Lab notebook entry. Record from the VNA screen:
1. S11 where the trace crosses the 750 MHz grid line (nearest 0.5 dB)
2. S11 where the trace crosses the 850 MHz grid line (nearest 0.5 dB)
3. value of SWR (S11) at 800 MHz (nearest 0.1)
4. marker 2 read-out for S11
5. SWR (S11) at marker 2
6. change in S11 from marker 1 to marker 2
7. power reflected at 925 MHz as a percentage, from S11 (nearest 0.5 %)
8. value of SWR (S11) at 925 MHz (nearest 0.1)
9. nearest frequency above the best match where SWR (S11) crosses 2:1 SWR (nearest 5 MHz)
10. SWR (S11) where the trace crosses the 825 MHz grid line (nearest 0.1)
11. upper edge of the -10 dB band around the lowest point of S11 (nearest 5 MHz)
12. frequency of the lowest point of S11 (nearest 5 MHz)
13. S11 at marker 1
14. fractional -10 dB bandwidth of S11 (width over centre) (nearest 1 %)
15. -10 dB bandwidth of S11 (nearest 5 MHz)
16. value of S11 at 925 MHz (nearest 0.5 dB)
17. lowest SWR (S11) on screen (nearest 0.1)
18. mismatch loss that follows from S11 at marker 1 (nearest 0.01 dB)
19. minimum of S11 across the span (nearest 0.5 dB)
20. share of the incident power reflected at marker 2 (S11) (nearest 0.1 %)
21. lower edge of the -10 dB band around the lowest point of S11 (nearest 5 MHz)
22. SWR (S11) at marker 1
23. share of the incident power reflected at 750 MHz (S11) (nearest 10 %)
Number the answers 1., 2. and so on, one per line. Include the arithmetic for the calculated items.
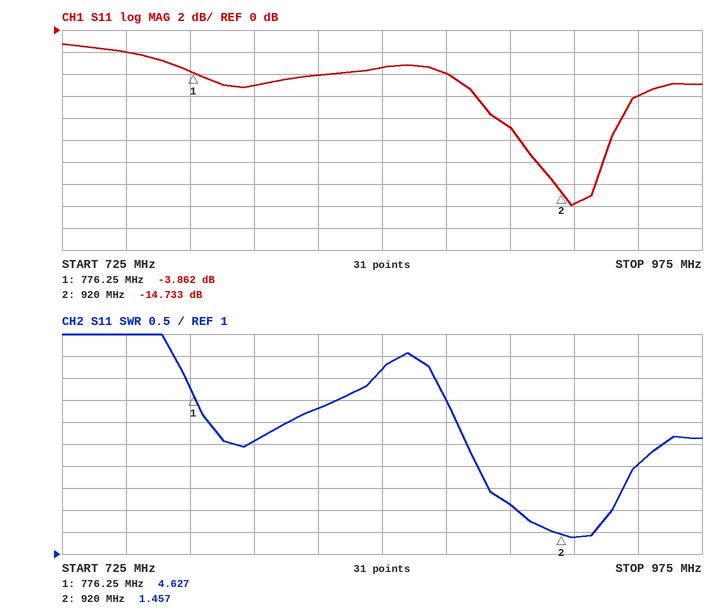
1. -2.0 dB
2. -3.5 dB
3. 3.6
4. -14.733 dB
5. 1.457
6. -14.733 − (-3.862) = -10.871 dB
7. 10^(-16/10) ≈ 2.5 %
8. 1.4
9. 940 MHz
10. 4.3
11. 940 MHz
12. 925 MHz
13. -3.862 dB
14. 35 MHz / 922.5 MHz ≈ 4 %
15. 940 MHz − 905 MHz = 35 MHz
16. -16.0 dB
17. 1.4
18. −10 log10(1 − 10^(-3.862/10)) ≈ 2.30 dB
19. -16.0 dB
20. 10^(-14.733/10) ≈ 3.4 %
21. 905 MHz
22. 4.627
23. 10^(-2/10) ≈ 63.1 %, so 60 % to the nearest 10 %
